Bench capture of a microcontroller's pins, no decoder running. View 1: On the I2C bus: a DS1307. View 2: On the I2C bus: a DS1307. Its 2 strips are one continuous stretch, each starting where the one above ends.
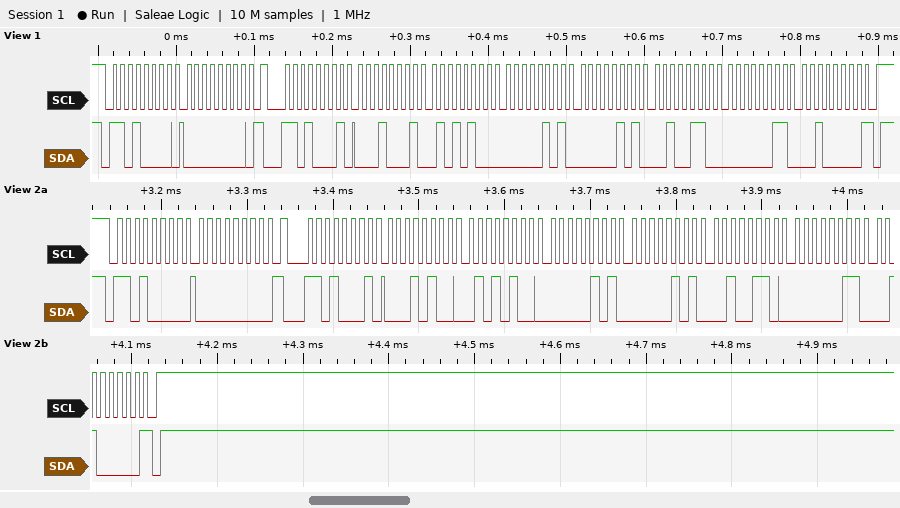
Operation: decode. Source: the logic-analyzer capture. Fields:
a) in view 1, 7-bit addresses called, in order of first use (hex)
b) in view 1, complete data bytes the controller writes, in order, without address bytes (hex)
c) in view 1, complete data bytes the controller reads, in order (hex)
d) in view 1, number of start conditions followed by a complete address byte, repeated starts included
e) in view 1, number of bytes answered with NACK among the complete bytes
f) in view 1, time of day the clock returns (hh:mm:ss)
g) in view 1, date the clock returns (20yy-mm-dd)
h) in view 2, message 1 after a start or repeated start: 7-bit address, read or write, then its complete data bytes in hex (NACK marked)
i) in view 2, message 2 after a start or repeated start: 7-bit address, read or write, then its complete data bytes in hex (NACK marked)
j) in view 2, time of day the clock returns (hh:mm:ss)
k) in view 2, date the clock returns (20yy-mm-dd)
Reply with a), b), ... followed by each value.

a) 0x68
b) 00
c) 11 54 05 05 26 03 20
d) 2
e) 1
f) 05:54:11
g) 2020-03-26
h) 0x68 write: 00
i) 0x68 read: 14 54 05 05 26 03 20 NACK
j) 05:54:14
k) 2020-03-26
